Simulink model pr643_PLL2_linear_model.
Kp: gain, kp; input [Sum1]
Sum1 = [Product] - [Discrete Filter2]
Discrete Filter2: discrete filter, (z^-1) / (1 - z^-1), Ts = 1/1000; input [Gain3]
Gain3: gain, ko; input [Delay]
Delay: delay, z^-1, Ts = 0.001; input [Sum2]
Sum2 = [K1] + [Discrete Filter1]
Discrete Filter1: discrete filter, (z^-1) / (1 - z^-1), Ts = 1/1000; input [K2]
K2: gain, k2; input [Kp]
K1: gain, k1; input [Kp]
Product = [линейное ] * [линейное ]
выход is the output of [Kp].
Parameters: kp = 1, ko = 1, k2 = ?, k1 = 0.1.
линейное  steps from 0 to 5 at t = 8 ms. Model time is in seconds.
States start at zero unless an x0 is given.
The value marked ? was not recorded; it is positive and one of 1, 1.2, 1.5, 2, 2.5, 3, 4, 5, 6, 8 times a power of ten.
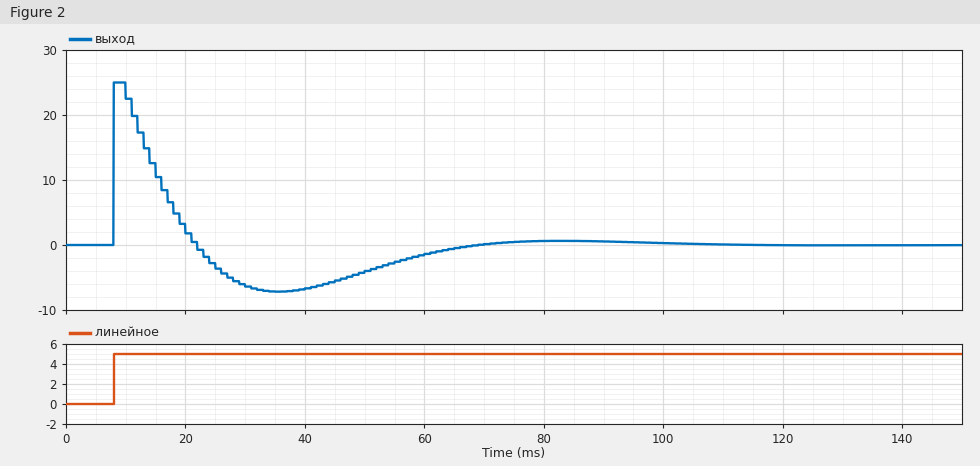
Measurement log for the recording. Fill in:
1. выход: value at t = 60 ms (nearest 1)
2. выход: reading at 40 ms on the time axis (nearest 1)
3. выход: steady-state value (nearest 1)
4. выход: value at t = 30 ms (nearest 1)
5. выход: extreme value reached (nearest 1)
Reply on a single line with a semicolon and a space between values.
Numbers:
-1; -7; 0; -6; 25
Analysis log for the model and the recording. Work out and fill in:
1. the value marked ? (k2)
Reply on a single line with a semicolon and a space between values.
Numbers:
0.006
